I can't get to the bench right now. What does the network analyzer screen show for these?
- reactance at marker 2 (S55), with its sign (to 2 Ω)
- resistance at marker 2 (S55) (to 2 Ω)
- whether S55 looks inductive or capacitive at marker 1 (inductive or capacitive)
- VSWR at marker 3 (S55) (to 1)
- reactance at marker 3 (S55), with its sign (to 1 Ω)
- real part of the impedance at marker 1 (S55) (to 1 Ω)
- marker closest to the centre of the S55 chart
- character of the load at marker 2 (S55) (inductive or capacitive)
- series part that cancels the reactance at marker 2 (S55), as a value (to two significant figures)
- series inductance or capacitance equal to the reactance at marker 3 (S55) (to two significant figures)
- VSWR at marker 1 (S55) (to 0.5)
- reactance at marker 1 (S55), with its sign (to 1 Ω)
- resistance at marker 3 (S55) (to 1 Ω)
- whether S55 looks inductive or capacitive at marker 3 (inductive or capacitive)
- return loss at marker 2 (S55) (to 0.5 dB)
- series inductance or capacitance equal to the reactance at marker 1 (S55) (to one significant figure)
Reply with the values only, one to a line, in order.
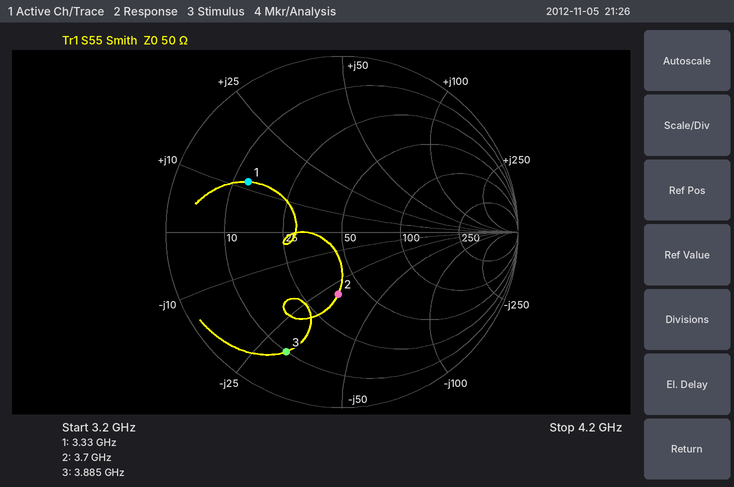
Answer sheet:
-30 Ω
38 Ω
inductive
7
-31 Ω
13 Ω
marker 2
capacitive
1.3 nH
1.3 pF
4.0
+12 Ω
10 Ω
capacitive
9.0 dB
600 pH
